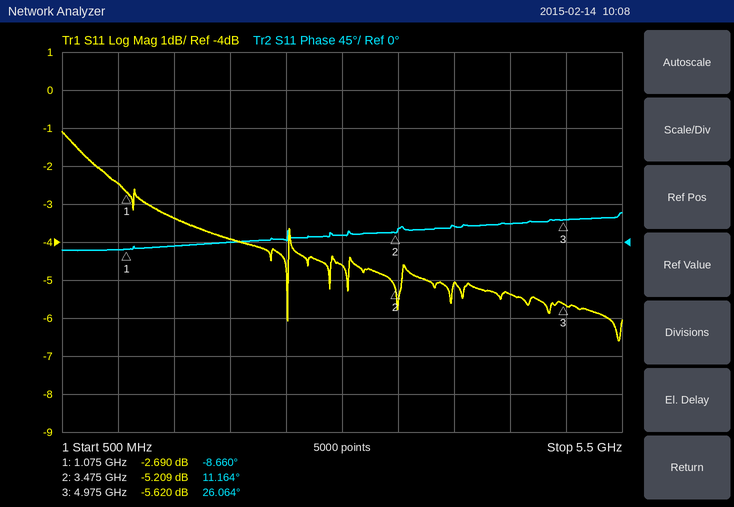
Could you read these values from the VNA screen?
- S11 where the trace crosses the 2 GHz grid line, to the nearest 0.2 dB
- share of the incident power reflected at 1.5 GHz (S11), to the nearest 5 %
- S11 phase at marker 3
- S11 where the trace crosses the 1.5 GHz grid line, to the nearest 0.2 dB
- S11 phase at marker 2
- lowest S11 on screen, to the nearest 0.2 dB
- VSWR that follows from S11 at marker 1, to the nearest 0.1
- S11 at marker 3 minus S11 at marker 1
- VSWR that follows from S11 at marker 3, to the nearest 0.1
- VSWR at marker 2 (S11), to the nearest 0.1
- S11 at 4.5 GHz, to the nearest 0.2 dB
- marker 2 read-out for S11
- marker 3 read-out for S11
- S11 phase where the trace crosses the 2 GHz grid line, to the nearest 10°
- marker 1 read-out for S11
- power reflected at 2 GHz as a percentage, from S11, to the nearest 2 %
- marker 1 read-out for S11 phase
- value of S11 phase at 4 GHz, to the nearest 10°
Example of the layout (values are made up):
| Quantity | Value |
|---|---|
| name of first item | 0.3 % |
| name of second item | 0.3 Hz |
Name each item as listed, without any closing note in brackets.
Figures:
| Quantity | Value |
|---|---|
| S11 where the trace crosses the 2 GHz grid line, to the nearest 0.2 dB | -4.0 dB |
| share of the incident power reflected at 1.5 GHz (S11), to the nearest 5 % | 45 % |
| S11 phase at marker 3 | 26.064° |
| S11 where the trace crosses the 1.5 GHz grid line, to the nearest 0.2 dB | -3.4 dB |
| S11 phase at marker 2 | 11.164° |
| lowest S11 on screen, to the nearest 0.2 dB | -6.6 dB |
| VSWR that follows from S11 at marker 1, to the nearest 0.1 | 6.5 |
| S11 at marker 3 minus S11 at marker 1 | -2.930 dB |
| VSWR that follows from S11 at marker 3, to the nearest 0.1 | 3.2 |
| VSWR at marker 2 (S11), to the nearest 0.1 | 3.4 |
| S11 at 4.5 GHz, to the nearest 0.2 dB | -5.4 dB |
| marker 2 read-out for S11 | -5.209 dB |
| marker 3 read-out for S11 | -5.620 dB |
| S11 phase where the trace crosses the 2 GHz grid line, to the nearest 10° | 0° |
| marker 1 read-out for S11 | -2.690 dB |
| power reflected at 2 GHz as a percentage, from S11, to the nearest 2 % | 40 % |
| marker 1 read-out for S11 phase | -8.660° |
| value of S11 phase at 4 GHz, to the nearest 10° | 20° |
